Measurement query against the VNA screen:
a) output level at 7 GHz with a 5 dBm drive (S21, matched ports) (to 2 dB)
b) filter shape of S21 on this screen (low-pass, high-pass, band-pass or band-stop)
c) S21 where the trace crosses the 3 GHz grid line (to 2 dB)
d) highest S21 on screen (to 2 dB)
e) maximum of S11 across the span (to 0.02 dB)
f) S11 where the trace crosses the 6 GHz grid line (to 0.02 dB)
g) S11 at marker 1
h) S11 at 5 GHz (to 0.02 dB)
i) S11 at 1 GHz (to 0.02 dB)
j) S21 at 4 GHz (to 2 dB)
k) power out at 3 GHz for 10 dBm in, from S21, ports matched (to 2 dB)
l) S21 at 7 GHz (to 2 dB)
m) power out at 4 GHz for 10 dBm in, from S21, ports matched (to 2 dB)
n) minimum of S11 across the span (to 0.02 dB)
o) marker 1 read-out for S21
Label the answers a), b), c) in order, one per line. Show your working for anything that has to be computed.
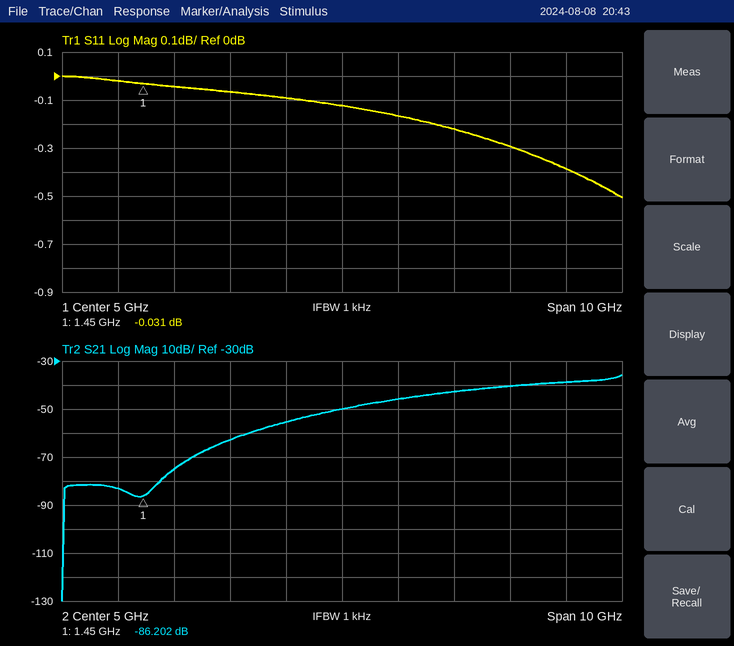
a) 5 dBm + (-42 dB) = -38 dBm
b) high-pass
c) -62 dB
d) -36 dB
e) 0.00 dB
f) -0.16 dB
g) -0.031 dB
h) -0.12 dB
i) -0.02 dB
j) -56 dB
k) 10 dBm + (-62 dB) = -52 dBm
l) -42 dB
m) 10 dBm + (-56 dB) = -46 dBm
n) -0.50 dB
o) -86.202 dB
